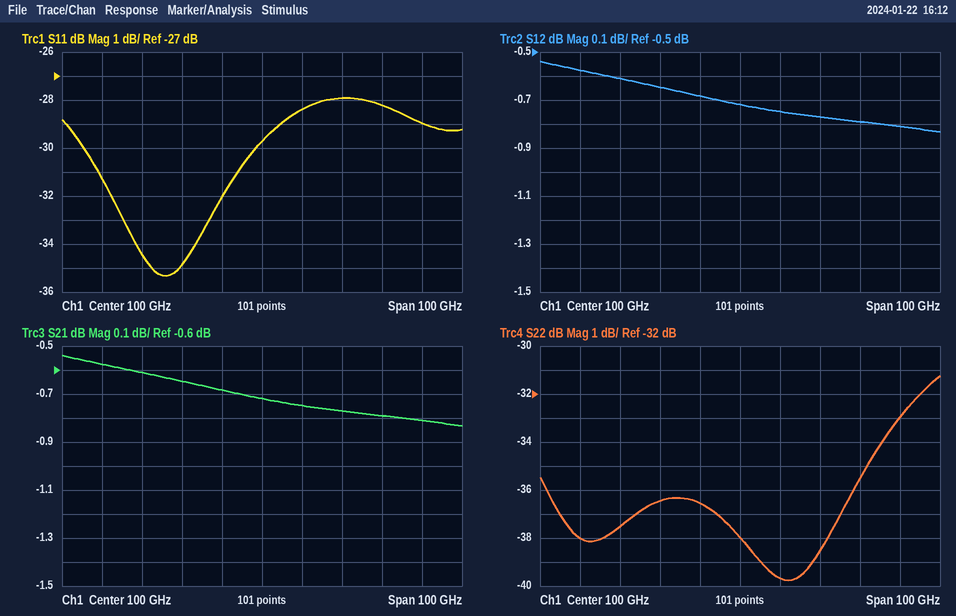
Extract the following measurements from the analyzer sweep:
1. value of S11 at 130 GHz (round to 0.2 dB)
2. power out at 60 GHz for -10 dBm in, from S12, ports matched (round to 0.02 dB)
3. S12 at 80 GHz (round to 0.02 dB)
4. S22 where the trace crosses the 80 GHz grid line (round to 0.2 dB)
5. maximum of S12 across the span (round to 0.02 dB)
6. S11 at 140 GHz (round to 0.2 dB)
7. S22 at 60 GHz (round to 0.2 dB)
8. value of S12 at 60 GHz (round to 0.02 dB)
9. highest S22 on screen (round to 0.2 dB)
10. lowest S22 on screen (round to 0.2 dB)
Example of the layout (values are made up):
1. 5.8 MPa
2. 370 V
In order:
1. -28.2 dB
2. -10.58 dBm
3. -0.64 dB
4. -36.4 dB
5. -0.54 dB
6. -29.0 dB
7. -38.0 dB
8. -0.58 dB
9. -31.2 dB
10. -39.8 dB
